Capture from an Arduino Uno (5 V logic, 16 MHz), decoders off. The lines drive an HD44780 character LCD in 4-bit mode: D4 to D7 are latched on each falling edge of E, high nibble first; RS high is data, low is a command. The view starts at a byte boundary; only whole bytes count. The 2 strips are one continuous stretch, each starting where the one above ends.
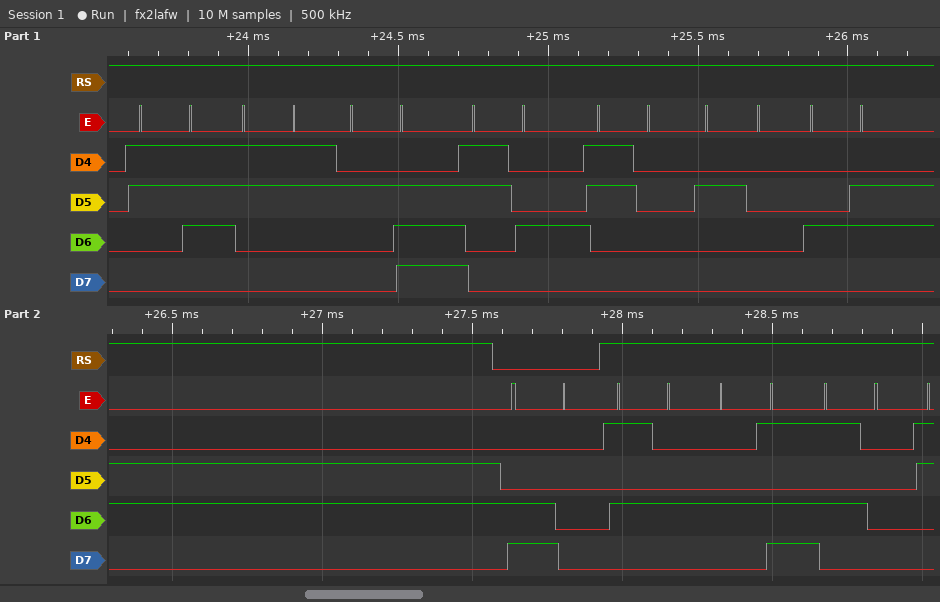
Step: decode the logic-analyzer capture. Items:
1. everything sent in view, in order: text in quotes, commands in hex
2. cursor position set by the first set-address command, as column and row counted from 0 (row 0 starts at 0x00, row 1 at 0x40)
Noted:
"73.40 F" 0xC0 "TMP"
column 0, row 1
